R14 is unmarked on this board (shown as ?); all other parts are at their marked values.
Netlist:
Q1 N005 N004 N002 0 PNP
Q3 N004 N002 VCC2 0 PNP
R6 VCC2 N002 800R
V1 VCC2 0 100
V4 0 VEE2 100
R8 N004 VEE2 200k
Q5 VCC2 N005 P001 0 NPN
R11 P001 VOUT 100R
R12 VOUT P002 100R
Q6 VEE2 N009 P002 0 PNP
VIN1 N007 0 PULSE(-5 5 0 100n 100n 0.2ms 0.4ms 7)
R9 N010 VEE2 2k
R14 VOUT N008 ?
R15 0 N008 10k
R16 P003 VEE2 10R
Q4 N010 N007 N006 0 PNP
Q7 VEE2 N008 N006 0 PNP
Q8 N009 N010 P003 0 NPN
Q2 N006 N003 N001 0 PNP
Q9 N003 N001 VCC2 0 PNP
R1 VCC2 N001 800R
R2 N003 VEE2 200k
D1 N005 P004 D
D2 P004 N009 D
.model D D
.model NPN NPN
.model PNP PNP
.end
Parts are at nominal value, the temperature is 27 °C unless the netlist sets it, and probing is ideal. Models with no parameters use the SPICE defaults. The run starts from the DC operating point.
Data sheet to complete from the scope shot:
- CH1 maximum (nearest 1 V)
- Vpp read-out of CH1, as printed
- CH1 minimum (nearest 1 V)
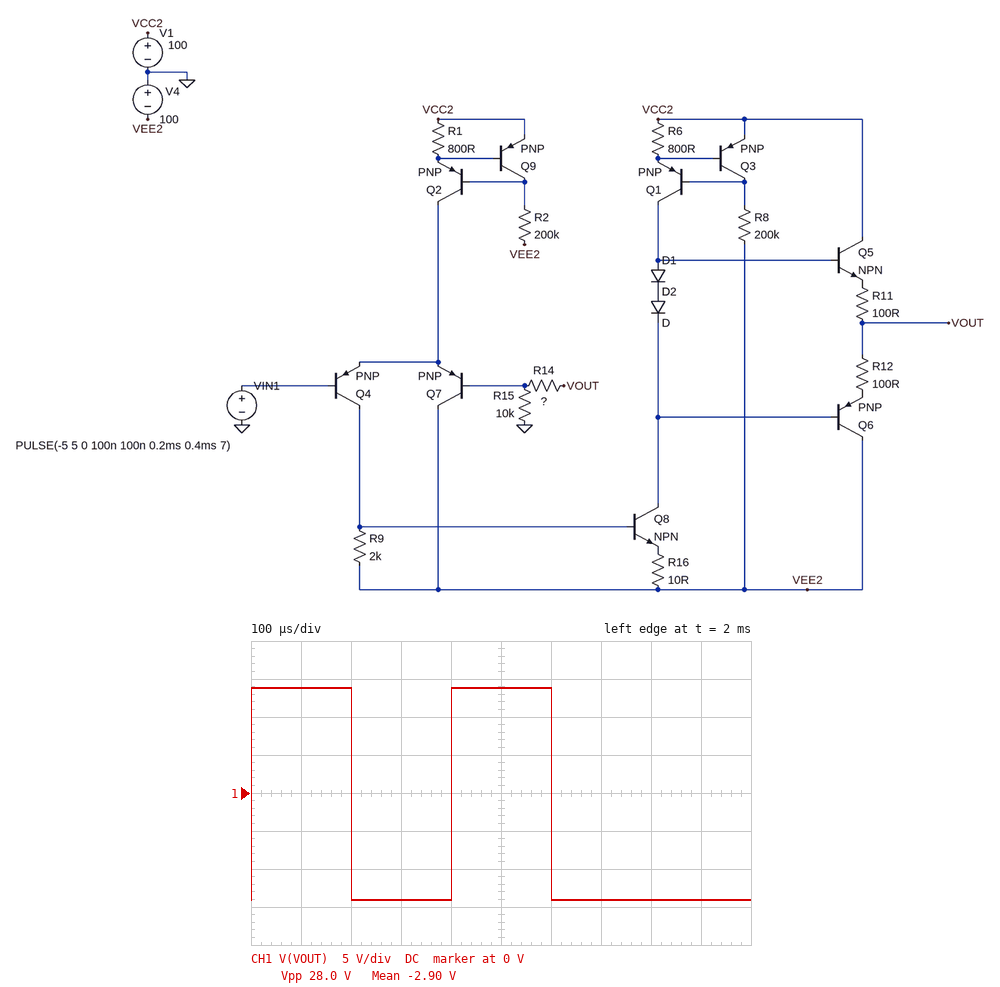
14 V
28.0 V
-14 V
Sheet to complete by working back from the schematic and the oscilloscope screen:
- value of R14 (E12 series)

18 kΩ
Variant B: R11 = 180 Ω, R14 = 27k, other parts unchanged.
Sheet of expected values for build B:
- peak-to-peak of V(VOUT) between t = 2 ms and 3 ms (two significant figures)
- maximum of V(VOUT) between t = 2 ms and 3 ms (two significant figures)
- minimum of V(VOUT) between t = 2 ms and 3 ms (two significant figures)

37 V
18 V
-19 V
